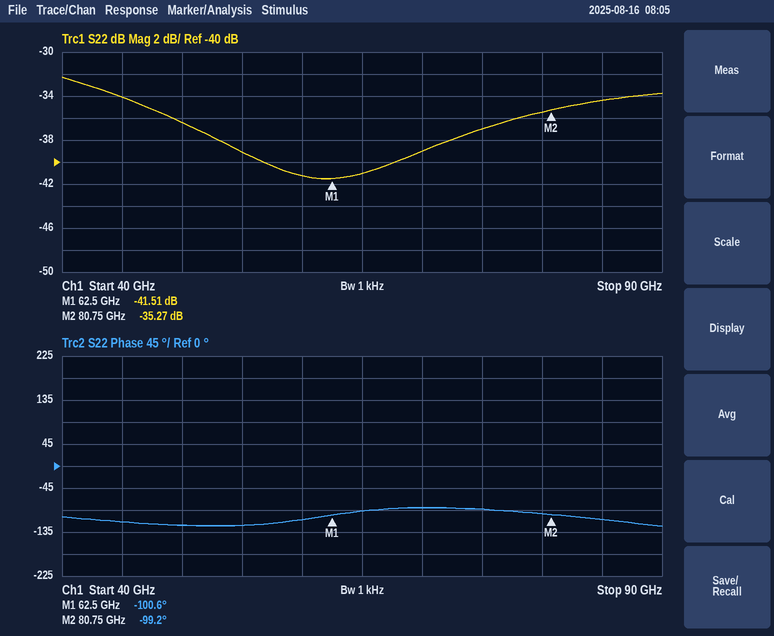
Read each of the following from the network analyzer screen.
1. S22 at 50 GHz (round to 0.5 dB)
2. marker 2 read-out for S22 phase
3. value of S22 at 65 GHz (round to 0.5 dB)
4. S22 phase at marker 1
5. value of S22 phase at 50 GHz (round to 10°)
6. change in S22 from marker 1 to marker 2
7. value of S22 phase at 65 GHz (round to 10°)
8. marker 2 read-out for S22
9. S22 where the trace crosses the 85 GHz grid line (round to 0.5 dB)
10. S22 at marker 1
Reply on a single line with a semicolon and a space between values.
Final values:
-36.5 dB; -99.2°; -41.0 dB; -100.6°; -120°; 6.24 dB; -90°; -35.27 dB; -34.5 dB; -41.51 dB
